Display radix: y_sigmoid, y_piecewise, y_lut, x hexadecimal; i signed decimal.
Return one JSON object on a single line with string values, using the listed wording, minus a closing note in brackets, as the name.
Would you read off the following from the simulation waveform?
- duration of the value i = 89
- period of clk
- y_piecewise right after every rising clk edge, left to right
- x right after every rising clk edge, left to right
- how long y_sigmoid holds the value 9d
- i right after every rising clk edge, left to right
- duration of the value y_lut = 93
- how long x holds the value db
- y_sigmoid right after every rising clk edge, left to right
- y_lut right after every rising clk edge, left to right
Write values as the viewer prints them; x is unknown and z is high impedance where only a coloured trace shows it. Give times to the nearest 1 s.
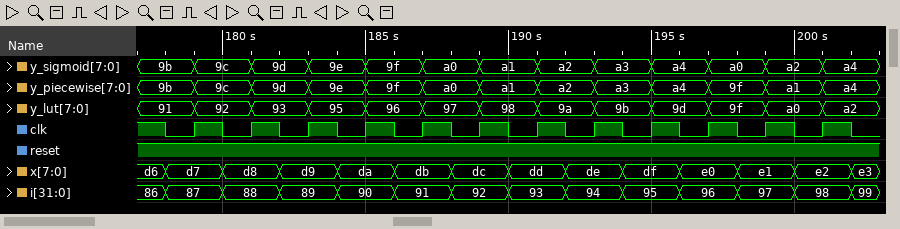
{"duration of the value i = 89": "2 s", "period of clk": "2 s", "y_piecewise right after every rising clk edge, left to right": "9c, 9d, 9e, 9f, a0, a1, a2, a3, a4, 9f, a1, a4", "x right after every rising clk edge, left to right": "d7, d8, d9, da, db, dc, dd, de, df, e0, e1, e2", "how long y_sigmoid holds the value 9d": "2 s", "i right after every rising clk edge, left to right": "87, 88, 89, 90, 91, 92, 93, 94, 95, 96, 97, 98", "duration of the value y_lut = 93": "2 s", "how long x holds the value db": "2 s", "y_sigmoid right after every rising clk edge, left to right": "9c, 9d, 9e, 9f, a0, a1, a2, a3, a4, a0, a2, a4", "y_lut right after every rising clk edge, left to right": "92, 93, 95, 96, 97, 98, 9a, 9b, 9d, 9f, a0, a2"}
